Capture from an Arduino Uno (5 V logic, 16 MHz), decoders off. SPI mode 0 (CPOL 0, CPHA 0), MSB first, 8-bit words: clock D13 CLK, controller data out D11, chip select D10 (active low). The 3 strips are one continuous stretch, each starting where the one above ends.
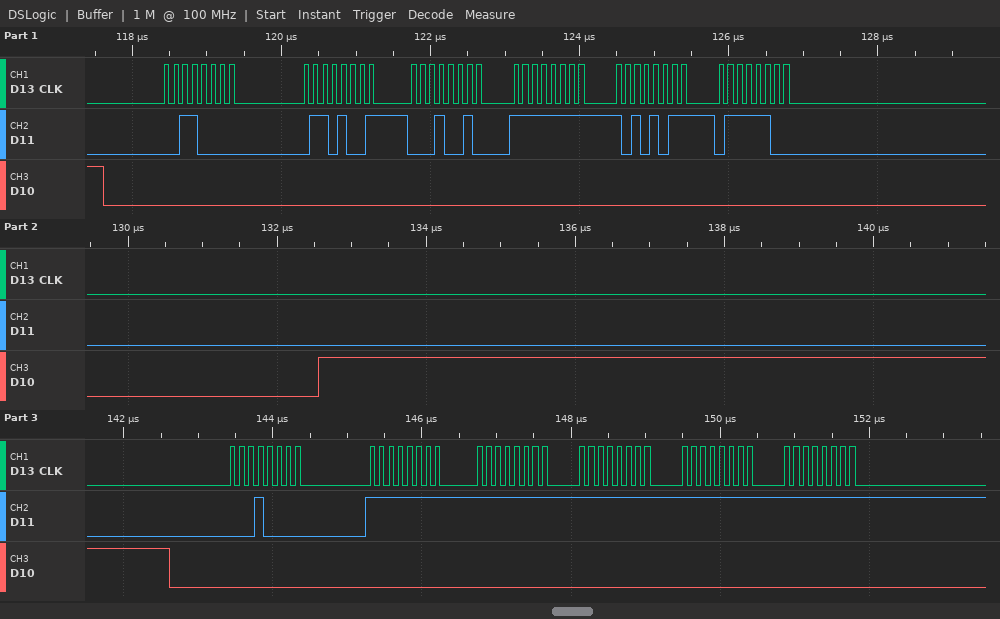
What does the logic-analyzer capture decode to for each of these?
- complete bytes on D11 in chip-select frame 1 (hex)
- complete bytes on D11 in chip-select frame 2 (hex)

30 69 12 FF AB 7C
10 FF FF FF FF FF
